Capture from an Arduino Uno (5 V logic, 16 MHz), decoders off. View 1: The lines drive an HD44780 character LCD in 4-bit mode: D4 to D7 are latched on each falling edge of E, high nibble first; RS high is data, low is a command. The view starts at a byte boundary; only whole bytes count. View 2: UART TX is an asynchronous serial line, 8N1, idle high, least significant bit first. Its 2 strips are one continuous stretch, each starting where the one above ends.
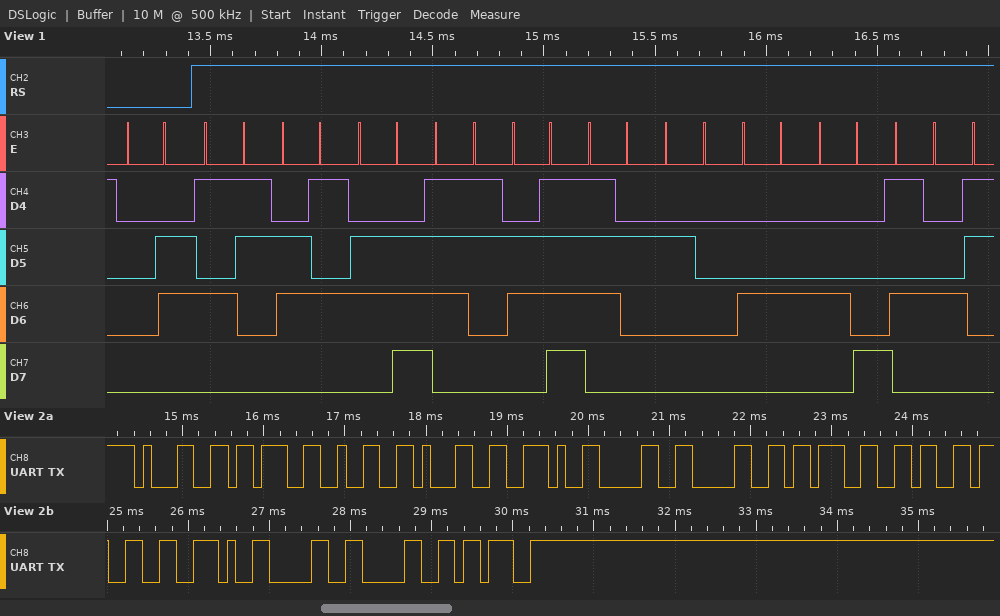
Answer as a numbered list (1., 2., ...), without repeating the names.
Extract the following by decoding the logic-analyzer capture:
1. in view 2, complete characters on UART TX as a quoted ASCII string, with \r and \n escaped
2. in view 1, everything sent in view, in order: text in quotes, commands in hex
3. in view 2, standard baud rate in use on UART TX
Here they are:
1. "1;21.00;63.00;"
2. 0x06 "Sensor DHT"
3. 9600 baud
